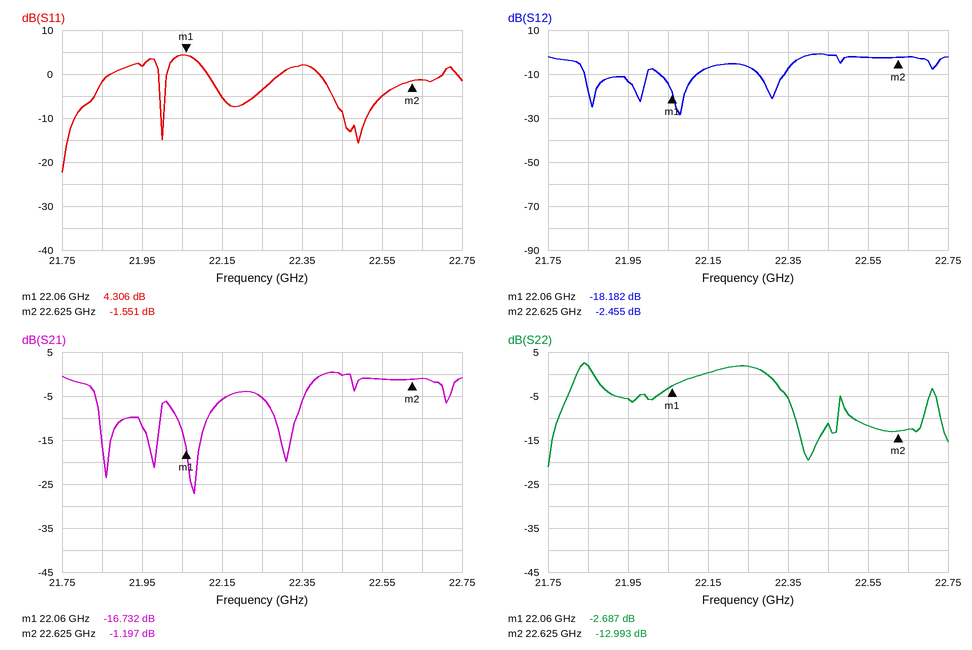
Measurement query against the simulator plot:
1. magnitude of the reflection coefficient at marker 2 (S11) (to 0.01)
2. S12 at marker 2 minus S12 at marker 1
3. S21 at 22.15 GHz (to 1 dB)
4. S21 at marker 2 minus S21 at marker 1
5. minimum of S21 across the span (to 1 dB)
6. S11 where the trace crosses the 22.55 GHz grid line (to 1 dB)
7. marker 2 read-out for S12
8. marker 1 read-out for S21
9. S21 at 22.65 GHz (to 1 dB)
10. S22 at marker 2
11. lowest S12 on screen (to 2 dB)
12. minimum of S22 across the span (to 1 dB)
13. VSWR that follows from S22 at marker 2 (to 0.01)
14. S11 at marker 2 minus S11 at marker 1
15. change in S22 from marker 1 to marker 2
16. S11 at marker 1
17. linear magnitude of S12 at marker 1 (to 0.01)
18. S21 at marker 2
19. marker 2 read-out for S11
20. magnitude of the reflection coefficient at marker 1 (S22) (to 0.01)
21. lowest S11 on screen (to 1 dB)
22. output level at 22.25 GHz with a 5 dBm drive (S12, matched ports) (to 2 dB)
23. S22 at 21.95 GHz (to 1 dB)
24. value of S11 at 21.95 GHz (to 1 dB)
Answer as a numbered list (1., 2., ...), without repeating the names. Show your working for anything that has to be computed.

1. 10^(-1.551/20) ≈ 0.84
2. -2.455 − (-18.182) = 15.727 dB
3. -6 dB
4. -1.197 − (-16.732) = 15.535 dB
5. -27 dB
6. -5 dB
7. -2.455 dB
8. -16.732 dB
9. -1 dB
10. -12.993 dB
11. -28 dB
12. -21 dB
13. (1 + 0.2241)/(1 − 0.2241) ≈ 1.58
14. -1.551 − (4.306) = -5.857 dB
15. -12.993 − (-2.687) = -10.306 dB
16. 4.306 dB
17. 10^(-18.182/20) ≈ 0.12
18. -1.197 dB
19. -1.551 dB
20. 10^(-2.687/20) ≈ 0.73
21. -22 dB
22. 5 dBm + (-6 dB) = -2 dBm
23. -6 dB
24. 2 dB
